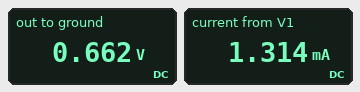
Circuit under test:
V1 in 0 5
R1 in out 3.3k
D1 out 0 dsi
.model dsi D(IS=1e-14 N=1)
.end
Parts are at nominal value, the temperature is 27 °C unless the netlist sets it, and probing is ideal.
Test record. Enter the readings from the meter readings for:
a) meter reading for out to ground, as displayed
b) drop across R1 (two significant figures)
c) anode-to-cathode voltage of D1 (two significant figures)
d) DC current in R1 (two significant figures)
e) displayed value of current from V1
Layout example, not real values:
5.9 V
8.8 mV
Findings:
0.662 V
4.3 V
660 mV
1.3 mA
1.314 mA
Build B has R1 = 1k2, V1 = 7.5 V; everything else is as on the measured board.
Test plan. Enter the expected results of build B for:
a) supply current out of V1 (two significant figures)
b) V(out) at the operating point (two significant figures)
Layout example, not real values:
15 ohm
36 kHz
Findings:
5.7 mA
700 mV
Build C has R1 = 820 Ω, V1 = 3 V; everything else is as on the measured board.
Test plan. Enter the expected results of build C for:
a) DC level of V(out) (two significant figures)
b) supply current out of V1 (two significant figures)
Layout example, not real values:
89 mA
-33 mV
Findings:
680 mV
2.8 mA
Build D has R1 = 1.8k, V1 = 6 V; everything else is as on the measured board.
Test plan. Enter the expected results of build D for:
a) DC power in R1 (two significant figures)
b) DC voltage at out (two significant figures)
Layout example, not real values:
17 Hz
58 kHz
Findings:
16 mW
680 mV
